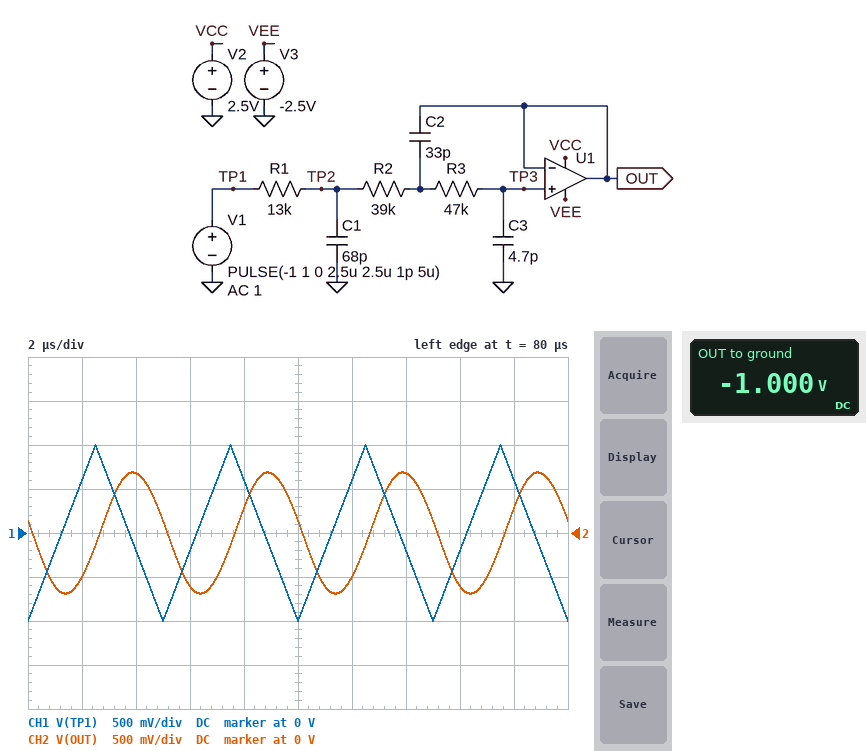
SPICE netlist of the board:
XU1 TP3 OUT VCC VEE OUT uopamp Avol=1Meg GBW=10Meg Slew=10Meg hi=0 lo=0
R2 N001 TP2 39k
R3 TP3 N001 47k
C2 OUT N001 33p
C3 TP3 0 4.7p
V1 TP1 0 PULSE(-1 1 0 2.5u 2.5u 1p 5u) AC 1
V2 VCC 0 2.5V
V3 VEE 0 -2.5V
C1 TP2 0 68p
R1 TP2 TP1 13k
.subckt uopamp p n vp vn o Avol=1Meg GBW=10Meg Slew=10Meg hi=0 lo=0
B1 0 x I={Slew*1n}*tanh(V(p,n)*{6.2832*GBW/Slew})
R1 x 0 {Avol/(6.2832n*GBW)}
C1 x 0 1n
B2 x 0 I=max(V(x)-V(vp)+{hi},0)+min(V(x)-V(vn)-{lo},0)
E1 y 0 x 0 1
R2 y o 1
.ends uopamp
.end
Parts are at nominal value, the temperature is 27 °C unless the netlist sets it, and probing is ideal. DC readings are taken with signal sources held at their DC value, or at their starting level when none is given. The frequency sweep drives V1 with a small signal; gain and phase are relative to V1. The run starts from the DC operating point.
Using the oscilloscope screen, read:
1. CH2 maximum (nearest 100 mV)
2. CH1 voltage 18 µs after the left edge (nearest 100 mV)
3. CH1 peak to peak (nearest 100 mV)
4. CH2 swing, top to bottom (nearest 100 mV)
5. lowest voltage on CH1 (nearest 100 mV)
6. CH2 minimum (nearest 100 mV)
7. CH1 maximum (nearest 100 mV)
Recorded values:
700 mV
600 mV
2.0 V
1.4 V
-1.0 V
-700 mV
1.0 V
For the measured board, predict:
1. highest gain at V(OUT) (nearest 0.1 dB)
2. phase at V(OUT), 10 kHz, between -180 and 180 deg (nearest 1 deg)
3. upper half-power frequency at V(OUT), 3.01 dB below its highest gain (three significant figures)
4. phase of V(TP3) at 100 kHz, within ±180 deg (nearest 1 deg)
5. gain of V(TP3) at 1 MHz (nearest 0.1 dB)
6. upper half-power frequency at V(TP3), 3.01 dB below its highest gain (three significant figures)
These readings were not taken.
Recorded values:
0 dB
-5 deg
253 kHz
-48 deg
-36.3 dB
253 kHz
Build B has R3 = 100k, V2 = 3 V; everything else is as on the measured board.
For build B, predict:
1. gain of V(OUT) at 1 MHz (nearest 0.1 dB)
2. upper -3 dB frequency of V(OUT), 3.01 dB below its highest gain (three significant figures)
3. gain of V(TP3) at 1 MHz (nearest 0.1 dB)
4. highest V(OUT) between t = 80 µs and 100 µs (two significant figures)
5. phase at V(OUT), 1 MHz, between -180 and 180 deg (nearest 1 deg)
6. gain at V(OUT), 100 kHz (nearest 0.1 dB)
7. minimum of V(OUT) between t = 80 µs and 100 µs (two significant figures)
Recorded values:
-42.9 dB
188 kHz
-42.8 dB
530 mV
108 deg
0.2 dB
-530 mV
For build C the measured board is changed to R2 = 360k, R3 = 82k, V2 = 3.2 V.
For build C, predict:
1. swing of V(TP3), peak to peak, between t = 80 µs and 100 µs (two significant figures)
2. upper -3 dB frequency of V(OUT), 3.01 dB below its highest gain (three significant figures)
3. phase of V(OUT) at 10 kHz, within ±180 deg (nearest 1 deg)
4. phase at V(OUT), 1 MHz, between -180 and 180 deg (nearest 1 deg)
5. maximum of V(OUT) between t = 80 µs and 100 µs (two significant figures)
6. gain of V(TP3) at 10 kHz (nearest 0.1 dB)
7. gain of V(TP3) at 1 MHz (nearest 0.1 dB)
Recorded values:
150 mV
81.4 kHz
-11 deg
99 deg
76 mV
0.1 dB
-60.5 dB
